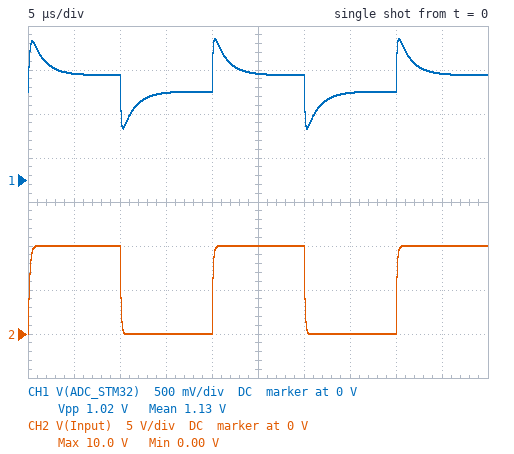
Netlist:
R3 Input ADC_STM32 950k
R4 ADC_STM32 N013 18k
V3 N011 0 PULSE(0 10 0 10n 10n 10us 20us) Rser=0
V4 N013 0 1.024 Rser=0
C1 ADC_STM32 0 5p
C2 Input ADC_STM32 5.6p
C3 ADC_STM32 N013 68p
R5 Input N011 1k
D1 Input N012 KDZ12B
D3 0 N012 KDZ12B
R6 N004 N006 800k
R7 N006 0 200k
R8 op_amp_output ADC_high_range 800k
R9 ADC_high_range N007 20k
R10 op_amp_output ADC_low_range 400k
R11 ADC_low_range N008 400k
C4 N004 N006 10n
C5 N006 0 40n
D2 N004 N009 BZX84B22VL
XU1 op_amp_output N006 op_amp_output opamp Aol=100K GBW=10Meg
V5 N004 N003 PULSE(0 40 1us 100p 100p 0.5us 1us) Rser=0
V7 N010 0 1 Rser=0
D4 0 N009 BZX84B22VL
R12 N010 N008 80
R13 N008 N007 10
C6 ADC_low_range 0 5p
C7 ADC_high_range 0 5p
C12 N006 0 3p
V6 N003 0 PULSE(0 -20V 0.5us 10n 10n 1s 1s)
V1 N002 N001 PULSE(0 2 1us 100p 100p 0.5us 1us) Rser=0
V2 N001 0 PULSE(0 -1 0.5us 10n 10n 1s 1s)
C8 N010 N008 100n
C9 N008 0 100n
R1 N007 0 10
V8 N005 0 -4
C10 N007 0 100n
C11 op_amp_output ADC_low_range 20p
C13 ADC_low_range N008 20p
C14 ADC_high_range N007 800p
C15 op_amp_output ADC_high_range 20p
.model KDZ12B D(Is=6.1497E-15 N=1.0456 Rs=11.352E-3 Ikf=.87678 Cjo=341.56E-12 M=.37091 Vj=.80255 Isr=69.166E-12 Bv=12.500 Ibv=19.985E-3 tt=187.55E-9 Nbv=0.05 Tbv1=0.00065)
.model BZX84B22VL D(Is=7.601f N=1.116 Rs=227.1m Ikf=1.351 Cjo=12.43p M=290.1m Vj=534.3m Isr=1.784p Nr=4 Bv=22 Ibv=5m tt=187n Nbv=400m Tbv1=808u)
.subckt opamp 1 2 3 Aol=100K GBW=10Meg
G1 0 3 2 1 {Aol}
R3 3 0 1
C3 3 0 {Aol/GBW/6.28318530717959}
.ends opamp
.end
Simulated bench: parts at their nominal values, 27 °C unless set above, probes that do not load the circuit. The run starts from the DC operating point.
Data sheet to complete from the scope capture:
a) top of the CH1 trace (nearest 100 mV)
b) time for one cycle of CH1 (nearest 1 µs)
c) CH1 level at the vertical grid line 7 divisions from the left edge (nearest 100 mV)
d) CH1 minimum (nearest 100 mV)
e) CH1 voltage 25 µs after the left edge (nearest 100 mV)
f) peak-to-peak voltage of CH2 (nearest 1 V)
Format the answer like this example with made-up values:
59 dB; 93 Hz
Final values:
1.6 V; 20 µs; 1.0 V; 600 mV; 1.2 V; 10 V
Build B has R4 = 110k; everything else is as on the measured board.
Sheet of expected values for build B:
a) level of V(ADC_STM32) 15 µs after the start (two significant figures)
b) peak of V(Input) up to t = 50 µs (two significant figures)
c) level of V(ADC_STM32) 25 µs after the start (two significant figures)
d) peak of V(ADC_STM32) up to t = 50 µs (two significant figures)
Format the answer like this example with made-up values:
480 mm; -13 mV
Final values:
1.0 V; 10 V; 1.8 V; 1.9 V
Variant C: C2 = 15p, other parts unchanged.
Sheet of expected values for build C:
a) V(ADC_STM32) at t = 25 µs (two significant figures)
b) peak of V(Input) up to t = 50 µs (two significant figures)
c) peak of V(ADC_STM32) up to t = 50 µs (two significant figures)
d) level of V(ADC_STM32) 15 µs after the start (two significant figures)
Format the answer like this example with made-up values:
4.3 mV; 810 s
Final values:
1.3 V; 10 V; 2.4 V; 940 mV
